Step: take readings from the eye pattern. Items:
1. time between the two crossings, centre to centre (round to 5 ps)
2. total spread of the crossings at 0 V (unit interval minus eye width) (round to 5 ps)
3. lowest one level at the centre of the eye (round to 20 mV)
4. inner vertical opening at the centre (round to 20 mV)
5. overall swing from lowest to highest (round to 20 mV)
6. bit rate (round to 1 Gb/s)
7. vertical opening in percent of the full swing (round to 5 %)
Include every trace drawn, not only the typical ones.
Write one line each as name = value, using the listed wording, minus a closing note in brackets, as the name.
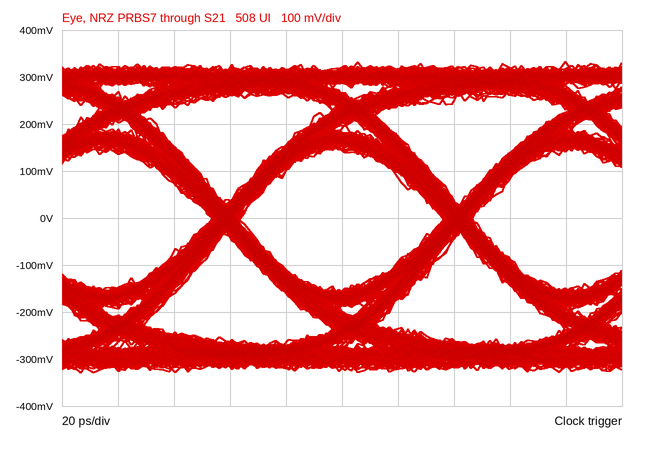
time between the two crossings, centre to centre = 85 ps
total spread of the crossings at 0 V (unit interval minus eye width) = 10 ps
lowest one level at the centre of the eye = 140 mV
inner vertical opening at the centre = 300 mV
overall swing from lowest to highest = 660 mV
bit rate = 12 Gb/s
vertical opening in percent of the full swing = 45 %
